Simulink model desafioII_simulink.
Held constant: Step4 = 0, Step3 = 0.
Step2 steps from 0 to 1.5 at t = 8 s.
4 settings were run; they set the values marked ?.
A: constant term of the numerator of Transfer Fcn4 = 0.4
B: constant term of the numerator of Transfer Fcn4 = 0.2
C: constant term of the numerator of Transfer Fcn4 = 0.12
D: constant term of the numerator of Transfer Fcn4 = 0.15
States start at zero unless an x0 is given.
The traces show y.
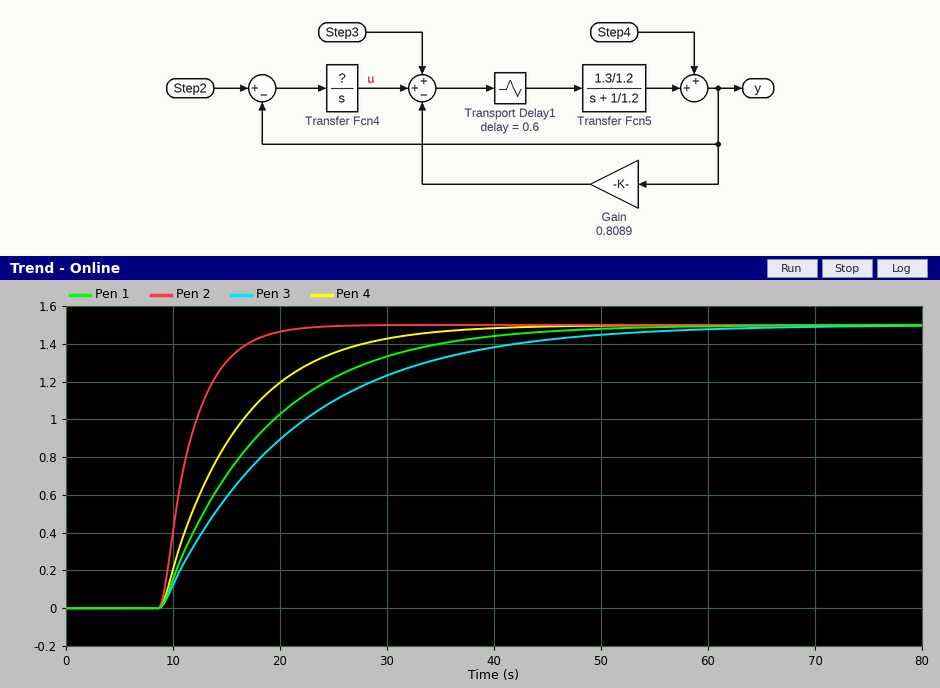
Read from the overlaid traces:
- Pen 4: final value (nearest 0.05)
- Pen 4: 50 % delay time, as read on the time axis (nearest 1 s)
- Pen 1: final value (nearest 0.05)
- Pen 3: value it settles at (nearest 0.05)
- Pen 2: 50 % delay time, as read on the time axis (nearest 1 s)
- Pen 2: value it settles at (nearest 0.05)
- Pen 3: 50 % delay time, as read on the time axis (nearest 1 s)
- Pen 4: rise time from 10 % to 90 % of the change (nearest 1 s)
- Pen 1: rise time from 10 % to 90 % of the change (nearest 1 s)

1.50
14 s
1.50
1.50
11 s
1.50
17 s
15 s
21 s
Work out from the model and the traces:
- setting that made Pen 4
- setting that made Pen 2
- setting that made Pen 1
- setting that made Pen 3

B
A
D
C
